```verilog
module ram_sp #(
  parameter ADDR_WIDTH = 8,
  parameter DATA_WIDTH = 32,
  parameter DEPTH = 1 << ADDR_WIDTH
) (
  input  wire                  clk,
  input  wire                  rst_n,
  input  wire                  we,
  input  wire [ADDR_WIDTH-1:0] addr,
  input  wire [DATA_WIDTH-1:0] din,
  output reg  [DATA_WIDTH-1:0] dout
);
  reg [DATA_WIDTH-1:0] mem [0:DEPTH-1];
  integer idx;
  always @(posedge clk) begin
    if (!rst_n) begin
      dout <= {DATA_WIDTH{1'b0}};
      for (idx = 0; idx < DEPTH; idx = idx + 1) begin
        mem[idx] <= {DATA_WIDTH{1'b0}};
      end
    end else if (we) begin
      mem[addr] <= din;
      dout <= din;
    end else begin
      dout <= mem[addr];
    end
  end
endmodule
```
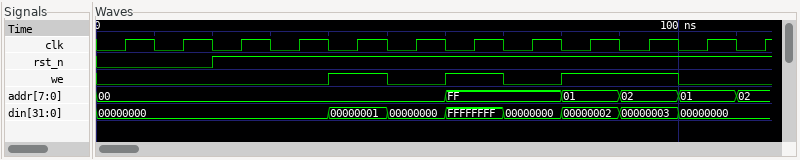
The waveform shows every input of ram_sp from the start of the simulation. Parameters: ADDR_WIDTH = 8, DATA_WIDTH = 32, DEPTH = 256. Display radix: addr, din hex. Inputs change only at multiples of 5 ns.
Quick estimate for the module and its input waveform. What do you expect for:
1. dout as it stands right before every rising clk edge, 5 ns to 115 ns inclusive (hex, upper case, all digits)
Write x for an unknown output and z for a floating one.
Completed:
x, 00000000, 00000000, 00000000, 00000000, 00000001, 00000001, FFFFFFFF, FFFFFFFF, 00000002, 00000003, 00000002
